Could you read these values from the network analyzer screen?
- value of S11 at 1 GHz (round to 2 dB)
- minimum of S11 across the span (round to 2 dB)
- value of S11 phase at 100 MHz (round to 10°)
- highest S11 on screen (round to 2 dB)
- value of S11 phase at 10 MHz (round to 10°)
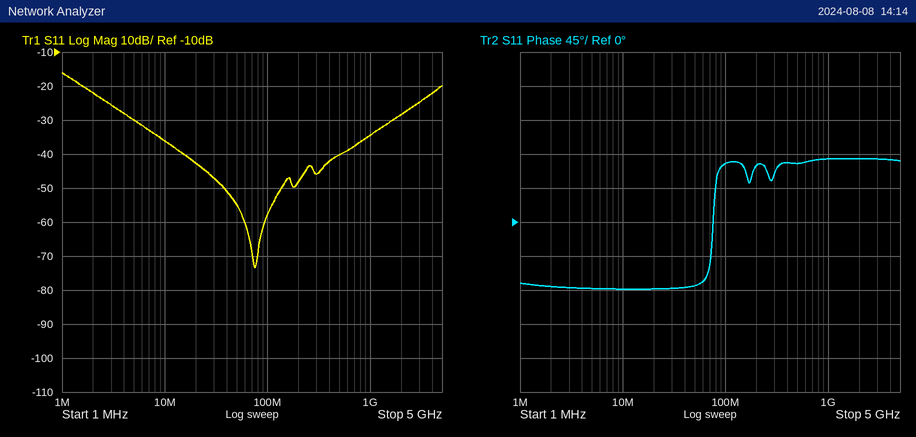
-34 dB
-74 dB
80°
-16 dB
-90°
